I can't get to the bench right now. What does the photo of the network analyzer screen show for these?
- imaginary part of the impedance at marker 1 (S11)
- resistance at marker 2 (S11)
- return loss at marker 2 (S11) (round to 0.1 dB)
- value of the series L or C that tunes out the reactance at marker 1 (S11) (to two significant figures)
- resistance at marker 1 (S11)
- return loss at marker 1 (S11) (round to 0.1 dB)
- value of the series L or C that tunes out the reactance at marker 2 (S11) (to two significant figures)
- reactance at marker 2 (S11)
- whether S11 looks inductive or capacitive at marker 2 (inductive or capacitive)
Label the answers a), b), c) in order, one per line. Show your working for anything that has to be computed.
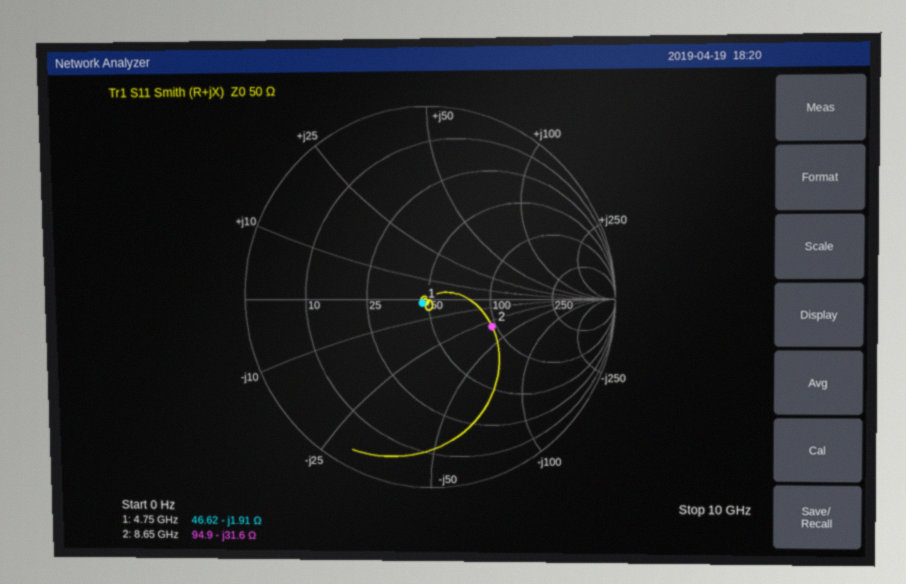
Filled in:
a) -1.91 Ω
b) 94.9 Ω
c) 8.6 dB
d) L = 1.91 Ω/(2π × 4.75 GHz) ≈ 64 pH
e) 46.62 Ω
f) 27.9 dB
g) L = 31.6 Ω/(2π × 8.65 GHz) ≈ 581 pH, so 580 pH to two significant figures
h) -31.6 Ω
i) capacitive
